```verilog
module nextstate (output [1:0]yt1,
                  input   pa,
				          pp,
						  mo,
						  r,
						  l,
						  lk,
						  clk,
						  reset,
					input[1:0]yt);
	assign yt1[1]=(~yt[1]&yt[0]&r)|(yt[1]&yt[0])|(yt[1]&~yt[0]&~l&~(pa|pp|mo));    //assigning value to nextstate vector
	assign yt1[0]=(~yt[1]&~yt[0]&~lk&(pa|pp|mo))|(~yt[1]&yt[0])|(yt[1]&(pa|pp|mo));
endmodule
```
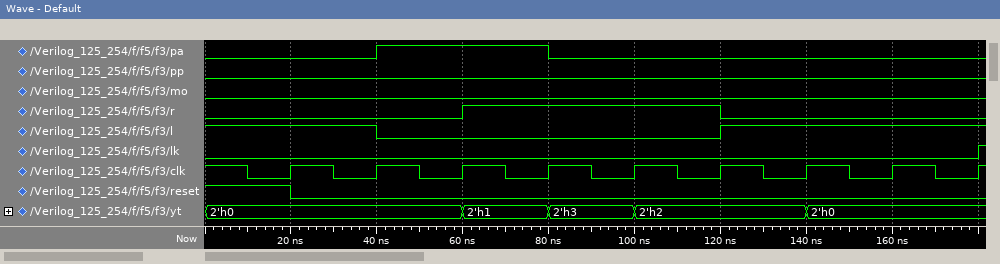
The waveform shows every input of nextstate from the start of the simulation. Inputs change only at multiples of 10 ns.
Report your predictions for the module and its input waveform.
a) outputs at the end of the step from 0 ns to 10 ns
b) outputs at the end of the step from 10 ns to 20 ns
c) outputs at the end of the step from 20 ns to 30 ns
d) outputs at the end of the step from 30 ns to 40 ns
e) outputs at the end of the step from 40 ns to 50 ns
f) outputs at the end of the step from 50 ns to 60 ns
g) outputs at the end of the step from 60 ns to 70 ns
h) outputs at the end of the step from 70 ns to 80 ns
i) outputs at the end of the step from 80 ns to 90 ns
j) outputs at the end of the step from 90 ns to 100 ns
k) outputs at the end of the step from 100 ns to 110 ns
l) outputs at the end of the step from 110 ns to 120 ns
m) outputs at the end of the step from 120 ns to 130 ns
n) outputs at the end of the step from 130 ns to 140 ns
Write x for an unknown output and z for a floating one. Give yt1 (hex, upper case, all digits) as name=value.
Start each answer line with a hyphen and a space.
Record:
- yt1=0
- yt1=0
- yt1=0
- yt1=0
- yt1=1
- yt1=1
- yt1=3
- yt1=3
- yt1=2
- yt1=2
- yt1=2
- yt1=2
- yt1=0
- yt1=0
